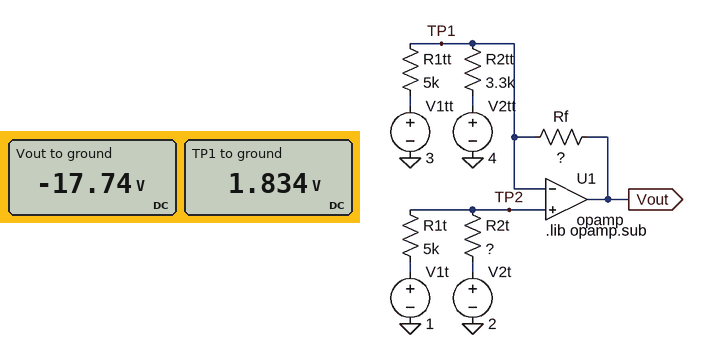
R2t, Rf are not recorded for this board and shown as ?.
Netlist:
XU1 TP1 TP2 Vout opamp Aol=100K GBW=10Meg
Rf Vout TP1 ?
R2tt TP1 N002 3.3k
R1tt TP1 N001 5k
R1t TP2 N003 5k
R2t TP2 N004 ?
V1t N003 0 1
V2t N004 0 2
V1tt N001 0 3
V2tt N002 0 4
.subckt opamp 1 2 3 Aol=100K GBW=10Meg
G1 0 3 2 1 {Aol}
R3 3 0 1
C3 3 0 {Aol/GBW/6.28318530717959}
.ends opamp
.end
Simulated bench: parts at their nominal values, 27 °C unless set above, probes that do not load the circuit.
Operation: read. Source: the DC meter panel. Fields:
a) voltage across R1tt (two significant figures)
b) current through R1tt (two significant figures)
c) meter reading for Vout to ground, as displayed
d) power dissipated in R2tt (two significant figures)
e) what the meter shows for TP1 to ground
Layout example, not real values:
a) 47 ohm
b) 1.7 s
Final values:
a) 1.2 V
b) 230 µA
c) -17.74 V
d) 1.4 mW
e) 1.834 V
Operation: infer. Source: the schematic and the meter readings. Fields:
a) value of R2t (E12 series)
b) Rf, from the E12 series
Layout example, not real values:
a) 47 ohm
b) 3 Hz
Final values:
a) 1 kΩ
b) 22 kΩ
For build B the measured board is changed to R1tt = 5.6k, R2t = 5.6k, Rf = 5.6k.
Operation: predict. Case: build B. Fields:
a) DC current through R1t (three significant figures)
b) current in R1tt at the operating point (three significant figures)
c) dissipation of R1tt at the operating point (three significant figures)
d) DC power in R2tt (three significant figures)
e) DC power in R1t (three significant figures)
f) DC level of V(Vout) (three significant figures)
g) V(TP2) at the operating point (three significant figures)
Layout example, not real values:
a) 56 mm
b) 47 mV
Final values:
a) 94.3 µA
b) 273 µA
c) 417 µW
d) 1.94 mW
e) 44.5 µW
f) -4.35 V
g) 1.47 V
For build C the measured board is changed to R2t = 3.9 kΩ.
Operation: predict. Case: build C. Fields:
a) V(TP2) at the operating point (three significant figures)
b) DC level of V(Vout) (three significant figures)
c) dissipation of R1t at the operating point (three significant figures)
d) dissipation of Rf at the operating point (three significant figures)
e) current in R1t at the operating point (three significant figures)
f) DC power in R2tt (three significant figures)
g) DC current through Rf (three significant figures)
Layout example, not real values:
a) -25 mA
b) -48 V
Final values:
a) 1.56 V
b) -21.0 V
c) 63.1 µW
d) 23.2 mW
e) 112 µA
f) 1.80 mW
g) 1.03 mA
